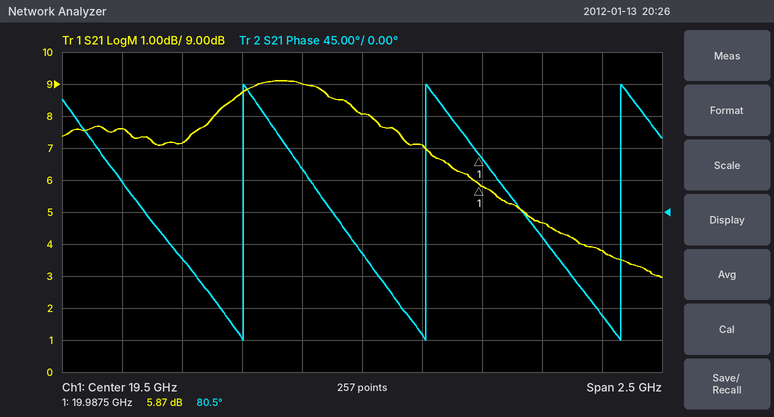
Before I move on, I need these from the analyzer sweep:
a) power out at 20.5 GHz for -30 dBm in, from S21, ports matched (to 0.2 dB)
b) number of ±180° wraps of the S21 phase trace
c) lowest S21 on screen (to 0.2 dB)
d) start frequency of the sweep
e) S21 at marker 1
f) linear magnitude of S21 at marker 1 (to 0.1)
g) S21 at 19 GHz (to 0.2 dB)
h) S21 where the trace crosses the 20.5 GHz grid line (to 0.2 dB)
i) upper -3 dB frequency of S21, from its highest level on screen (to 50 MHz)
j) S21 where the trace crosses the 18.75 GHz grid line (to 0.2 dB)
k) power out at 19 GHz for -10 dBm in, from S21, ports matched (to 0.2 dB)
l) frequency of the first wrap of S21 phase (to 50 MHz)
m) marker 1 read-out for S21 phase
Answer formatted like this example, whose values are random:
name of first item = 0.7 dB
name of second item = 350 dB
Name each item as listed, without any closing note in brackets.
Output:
power out at 20.5 GHz for -30 dBm in, from S21, ports matched = -26.2 dBm
number of ±180° wraps of the S21 phase trace = 3
lowest S21 on screen = 3.0 dB
start frequency of the sweep = 18.25 GHz
S21 at marker 1 = 5.87 dB
linear magnitude of S21 at marker 1 = 2.0
S21 at 19 GHz = 8.8 dB
S21 where the trace crosses the 20.5 GHz grid line = 3.8 dB
upper -3 dB frequency of S21, from its highest level on screen = 19.95 GHz
S21 where the trace crosses the 18.75 GHz grid line = 7.2 dB
power out at 19 GHz for -10 dBm in, from S21, ports matched = -1.2 dBm
frequency of the first wrap of S21 phase = 19.00 GHz
marker 1 read-out for S21 phase = 80.5°
